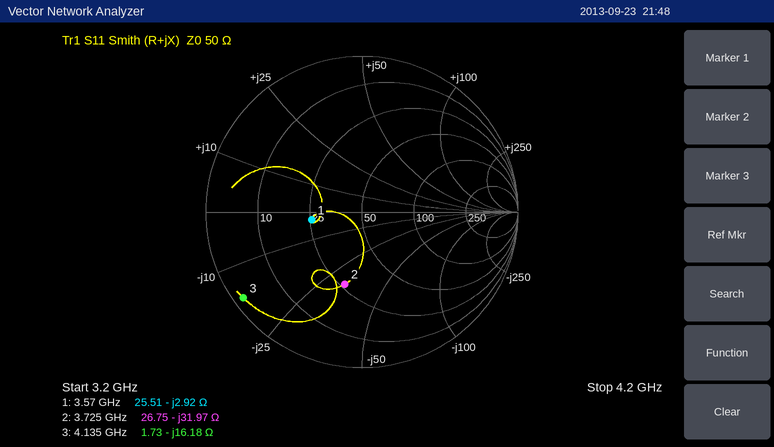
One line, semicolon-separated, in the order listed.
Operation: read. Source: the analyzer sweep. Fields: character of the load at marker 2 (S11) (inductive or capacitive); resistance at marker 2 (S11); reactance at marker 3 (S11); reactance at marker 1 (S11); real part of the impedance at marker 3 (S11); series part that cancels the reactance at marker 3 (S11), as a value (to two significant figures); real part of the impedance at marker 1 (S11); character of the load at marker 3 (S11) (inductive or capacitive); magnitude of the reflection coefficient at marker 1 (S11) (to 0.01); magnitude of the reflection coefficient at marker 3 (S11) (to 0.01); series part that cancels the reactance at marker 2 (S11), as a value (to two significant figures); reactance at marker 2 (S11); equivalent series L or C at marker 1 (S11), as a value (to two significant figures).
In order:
capacitive; 26.75 Ω; -16.18 Ω; -2.92 Ω; 1.73 Ω; 620 pH; 25.51 Ω; capacitive; 0.33; 0.94; 1.4 nH; -31.97 Ω; 15 pF
